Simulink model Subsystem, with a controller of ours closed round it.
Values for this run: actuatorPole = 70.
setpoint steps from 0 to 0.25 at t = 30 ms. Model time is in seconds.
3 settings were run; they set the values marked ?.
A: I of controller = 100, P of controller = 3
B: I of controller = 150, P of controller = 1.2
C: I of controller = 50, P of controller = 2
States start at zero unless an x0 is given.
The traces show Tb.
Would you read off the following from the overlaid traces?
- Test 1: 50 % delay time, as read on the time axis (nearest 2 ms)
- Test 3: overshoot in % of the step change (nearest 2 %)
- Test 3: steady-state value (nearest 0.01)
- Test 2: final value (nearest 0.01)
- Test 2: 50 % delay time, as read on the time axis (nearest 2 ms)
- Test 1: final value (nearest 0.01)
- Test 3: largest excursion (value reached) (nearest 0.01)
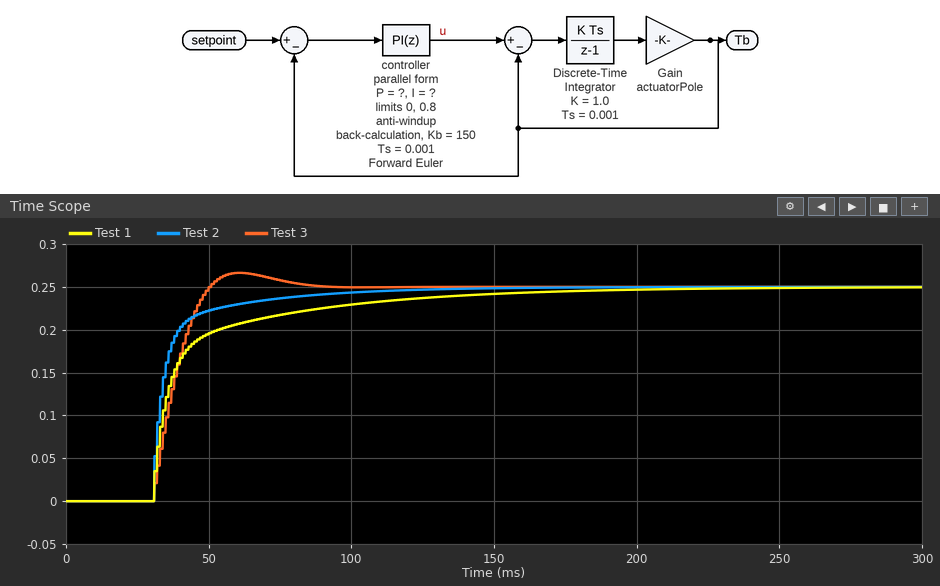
36 ms
6 %
0.25
0.25
34 ms
0.25
0.27
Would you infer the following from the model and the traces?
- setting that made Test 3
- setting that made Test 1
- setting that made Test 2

B
C
A
